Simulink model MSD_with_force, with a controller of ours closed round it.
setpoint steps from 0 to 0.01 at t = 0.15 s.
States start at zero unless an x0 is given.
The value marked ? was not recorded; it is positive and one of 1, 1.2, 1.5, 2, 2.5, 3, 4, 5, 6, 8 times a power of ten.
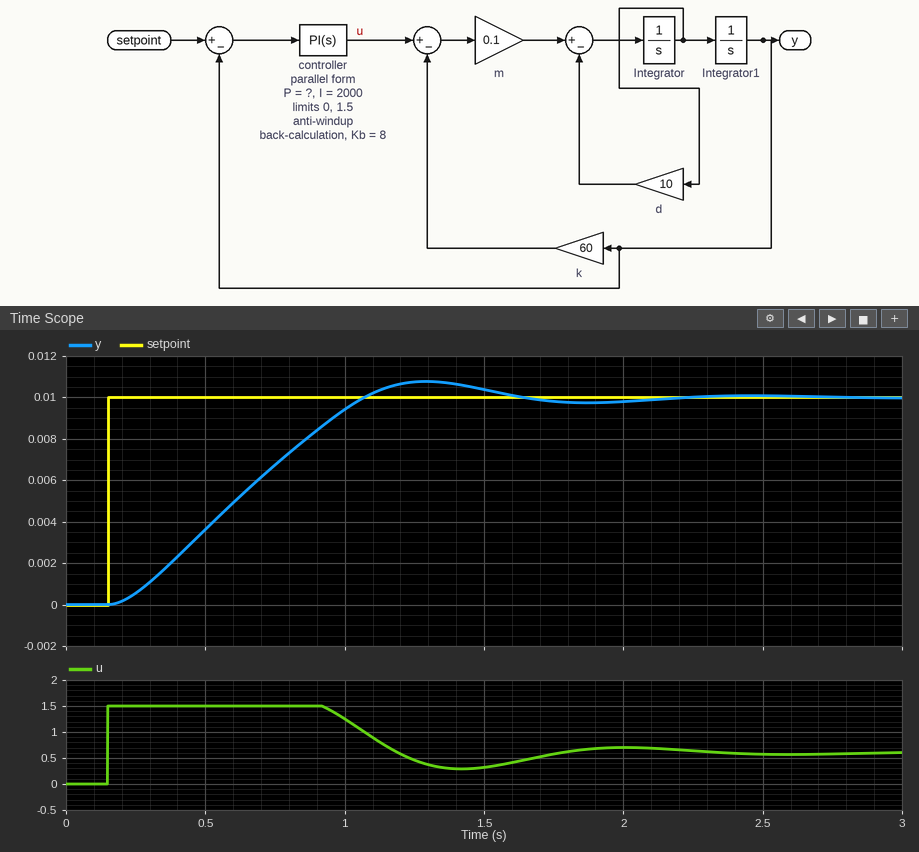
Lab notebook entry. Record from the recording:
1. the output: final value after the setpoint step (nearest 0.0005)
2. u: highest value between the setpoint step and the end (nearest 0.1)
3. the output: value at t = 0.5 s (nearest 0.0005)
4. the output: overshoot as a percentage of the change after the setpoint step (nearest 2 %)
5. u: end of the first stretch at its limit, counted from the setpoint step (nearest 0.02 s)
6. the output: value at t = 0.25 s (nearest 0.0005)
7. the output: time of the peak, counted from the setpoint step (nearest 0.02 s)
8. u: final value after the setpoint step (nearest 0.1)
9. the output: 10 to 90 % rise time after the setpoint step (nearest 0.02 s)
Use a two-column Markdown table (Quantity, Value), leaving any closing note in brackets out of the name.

| Quantity | Value |
|---|---|
| the output: final value after the setpoint step | 0.0100 |
| u: highest value between the setpoint step and the end | 1.5 |
| the output: value at t = 0.5 s | 0.0035 |
| the output: overshoot as a percentage of the change after the setpoint step | 8 % |
| u: end of the first stretch at its limit, counted from the setpoint step | 0.78 s |
| the output: value at t = 0.25 s | 0.0005 |
| the output: time of the peak, counted from the setpoint step | 1.14 s |
| u: final value after the setpoint step | 0.6 |
| the output: 10 to 90 % rise time after the setpoint step | 0.66 s |
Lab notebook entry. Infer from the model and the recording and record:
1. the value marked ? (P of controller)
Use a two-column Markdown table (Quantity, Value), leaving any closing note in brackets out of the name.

| Quantity | Value |
|---|---|
| the value marked ? | 500 |
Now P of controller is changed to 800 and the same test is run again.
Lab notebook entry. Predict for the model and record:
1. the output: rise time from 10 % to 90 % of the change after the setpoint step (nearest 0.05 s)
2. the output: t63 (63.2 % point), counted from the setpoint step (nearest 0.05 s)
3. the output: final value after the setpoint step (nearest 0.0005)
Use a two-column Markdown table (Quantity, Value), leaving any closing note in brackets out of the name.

| Quantity | Value |
|---|---|
| the output: rise time from 10 % to 90 % of the change after the setpoint step | 0.70 s |
| the output: t63 (63.2 % point), counted from the setpoint step | 0.55 s |
| the output: final value after the setpoint step | 0.0100 |
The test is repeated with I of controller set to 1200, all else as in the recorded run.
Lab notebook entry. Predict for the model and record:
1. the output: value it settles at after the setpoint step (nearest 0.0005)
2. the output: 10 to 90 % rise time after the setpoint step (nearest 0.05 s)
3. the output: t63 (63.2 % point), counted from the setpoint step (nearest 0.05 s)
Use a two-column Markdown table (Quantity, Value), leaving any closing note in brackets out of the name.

| Quantity | Value |
|---|---|
| the output: value it settles at after the setpoint step | 0.0100 |
| the output: 10 to 90 % rise time after the setpoint step | 0.70 s |
| the output: t63 (63.2 % point), counted from the setpoint step | 0.55 s |
